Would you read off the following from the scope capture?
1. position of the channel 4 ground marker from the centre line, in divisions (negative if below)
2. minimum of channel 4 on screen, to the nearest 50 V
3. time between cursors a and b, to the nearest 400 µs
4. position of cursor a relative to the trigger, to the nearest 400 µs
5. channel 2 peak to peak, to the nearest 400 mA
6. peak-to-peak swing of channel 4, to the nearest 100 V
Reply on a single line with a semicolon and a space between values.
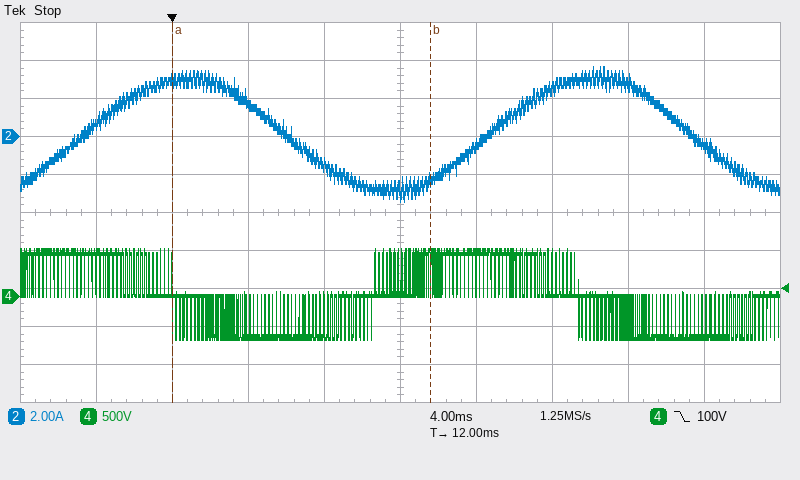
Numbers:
-2.2 div; -600 V; 13.6 ms; 0.0 ms; 7.2 A; 1.20 kV
